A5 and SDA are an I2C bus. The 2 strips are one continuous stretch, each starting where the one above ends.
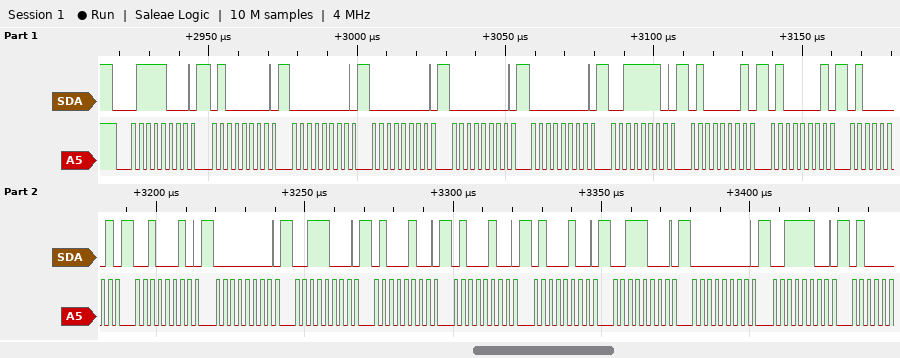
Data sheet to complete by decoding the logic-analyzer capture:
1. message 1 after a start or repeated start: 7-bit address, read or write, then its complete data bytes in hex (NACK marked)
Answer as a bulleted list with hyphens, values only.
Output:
- 0x3C write: 40 00 00 00 00 3E 41 41 41 22 00 38 44 44 44 38 00 3C
